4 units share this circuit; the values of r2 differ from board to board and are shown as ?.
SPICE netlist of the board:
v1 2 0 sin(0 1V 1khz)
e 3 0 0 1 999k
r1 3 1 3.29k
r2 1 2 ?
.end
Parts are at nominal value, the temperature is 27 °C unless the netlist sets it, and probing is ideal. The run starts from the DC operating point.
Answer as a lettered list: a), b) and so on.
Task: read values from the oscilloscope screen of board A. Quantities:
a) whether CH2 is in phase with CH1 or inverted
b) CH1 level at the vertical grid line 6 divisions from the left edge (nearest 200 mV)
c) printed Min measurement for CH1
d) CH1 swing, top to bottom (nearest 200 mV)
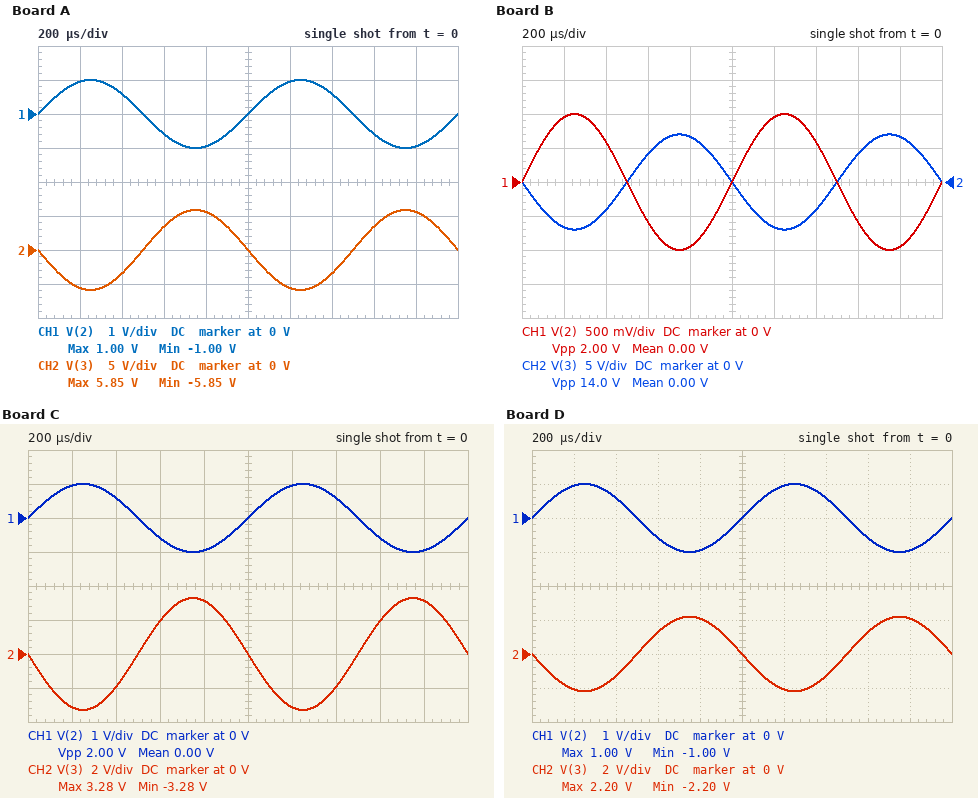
a) inverted
b) 1.0 V
c) -1.00 V
d) 2.0 V
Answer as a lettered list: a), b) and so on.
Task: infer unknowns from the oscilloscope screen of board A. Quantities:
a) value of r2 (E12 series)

a) 560 Ω
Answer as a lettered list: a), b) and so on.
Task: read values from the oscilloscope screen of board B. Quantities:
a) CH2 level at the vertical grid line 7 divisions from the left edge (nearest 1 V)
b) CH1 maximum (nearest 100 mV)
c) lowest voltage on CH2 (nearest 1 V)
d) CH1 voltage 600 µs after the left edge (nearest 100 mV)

a) -4 V
b) 1.0 V
c) -7 V
d) -600 mV
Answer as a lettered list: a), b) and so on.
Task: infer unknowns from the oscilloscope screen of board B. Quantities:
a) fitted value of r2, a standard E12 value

a) 470 Ω
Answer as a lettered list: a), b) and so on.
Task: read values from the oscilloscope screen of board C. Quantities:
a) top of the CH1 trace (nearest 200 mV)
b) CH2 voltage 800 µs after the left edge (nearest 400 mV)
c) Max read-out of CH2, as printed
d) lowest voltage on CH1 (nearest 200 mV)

a) 1.0 V
b) 3.2 V
c) 3.28 V
d) -1.0 V
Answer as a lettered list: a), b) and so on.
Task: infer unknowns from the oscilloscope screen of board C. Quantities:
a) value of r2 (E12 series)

a) 1 kΩ
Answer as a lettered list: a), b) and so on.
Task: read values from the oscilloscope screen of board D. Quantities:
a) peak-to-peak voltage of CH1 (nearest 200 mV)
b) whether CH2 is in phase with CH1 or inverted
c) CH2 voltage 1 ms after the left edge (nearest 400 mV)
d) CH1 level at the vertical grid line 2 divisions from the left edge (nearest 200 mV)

a) 2.0 V
b) inverted
c) 0 V
d) 600 mV
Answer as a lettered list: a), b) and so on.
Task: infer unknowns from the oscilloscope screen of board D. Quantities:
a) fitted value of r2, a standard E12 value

a) 1.5 kΩ
